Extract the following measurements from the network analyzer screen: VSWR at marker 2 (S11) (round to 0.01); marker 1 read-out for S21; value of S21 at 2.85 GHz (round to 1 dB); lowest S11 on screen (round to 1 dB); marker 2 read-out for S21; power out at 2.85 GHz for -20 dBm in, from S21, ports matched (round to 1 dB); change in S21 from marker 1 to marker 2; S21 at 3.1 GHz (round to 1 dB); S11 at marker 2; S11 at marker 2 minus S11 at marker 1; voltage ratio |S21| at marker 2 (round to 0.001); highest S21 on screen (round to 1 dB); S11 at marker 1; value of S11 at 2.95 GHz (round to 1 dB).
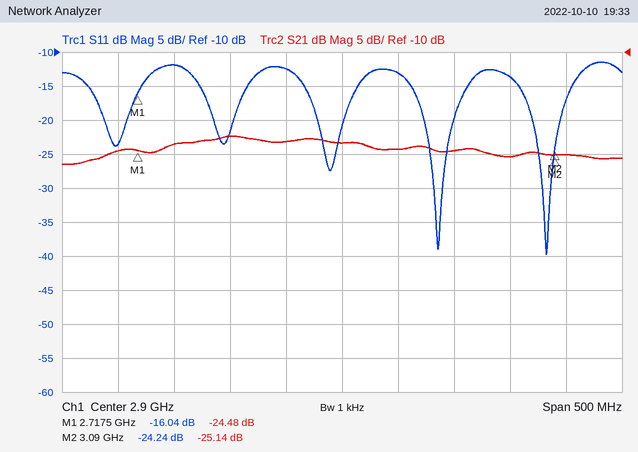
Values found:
1.13
-24.48 dB
-23 dB
-40 dB
-25.14 dB
-43 dBm
-0.66 dB
-25 dB
-24.24 dB
-8.20 dB
0.055
-22 dB
-16.04 dB
-13 dB
